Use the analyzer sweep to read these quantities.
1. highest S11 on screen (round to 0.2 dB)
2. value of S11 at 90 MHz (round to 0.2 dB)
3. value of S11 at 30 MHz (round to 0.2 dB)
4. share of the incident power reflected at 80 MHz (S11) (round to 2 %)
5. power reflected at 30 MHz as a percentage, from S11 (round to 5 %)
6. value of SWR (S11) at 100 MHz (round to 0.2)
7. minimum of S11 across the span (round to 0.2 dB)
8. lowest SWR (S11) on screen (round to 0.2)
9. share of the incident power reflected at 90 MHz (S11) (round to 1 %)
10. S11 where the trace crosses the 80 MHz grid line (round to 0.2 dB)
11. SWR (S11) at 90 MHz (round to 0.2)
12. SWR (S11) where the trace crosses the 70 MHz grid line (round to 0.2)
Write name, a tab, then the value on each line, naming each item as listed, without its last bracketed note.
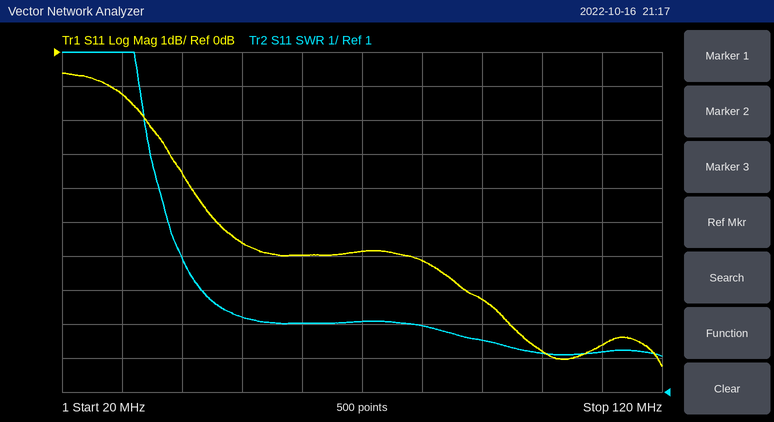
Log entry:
highest S11 on screen	-0.6 dB
value of S11 at 90 MHz	-7.2 dB
value of S11 at 30 MHz	-1.2 dB
share of the incident power reflected at 80 MHz (S11)	24 %
power reflected at 30 MHz as a percentage, from S11	75 %
value of SWR (S11) at 100 MHz	2.2
minimum of S11 across the span	-9.2 dB
lowest SWR (S11) on screen	2.0
share of the incident power reflected at 90 MHz (S11)	19 %
S11 where the trace crosses the 80 MHz grid line	-6.2 dB
SWR (S11) at 90 MHz	2.6
SWR (S11) where the trace crosses the 70 MHz grid line	3.0
